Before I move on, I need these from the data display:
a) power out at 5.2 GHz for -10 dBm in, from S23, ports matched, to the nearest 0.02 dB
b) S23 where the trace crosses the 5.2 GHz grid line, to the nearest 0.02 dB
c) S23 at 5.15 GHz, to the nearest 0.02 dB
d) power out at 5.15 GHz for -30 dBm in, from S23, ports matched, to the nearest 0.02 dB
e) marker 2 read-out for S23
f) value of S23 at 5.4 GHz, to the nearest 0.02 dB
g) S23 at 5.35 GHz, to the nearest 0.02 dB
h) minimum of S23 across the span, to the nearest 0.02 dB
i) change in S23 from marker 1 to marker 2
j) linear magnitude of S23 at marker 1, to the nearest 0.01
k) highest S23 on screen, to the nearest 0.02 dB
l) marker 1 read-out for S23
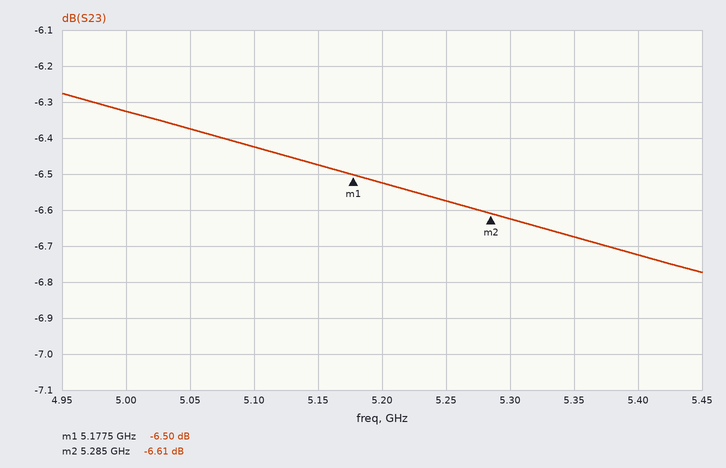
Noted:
-16.52 dBm
-6.52 dB
-6.48 dB
-36.48 dBm
-6.61 dB
-6.72 dB
-6.68 dB
-6.78 dB
-0.11 dB
0.47
-6.28 dB
-6.50 dB
